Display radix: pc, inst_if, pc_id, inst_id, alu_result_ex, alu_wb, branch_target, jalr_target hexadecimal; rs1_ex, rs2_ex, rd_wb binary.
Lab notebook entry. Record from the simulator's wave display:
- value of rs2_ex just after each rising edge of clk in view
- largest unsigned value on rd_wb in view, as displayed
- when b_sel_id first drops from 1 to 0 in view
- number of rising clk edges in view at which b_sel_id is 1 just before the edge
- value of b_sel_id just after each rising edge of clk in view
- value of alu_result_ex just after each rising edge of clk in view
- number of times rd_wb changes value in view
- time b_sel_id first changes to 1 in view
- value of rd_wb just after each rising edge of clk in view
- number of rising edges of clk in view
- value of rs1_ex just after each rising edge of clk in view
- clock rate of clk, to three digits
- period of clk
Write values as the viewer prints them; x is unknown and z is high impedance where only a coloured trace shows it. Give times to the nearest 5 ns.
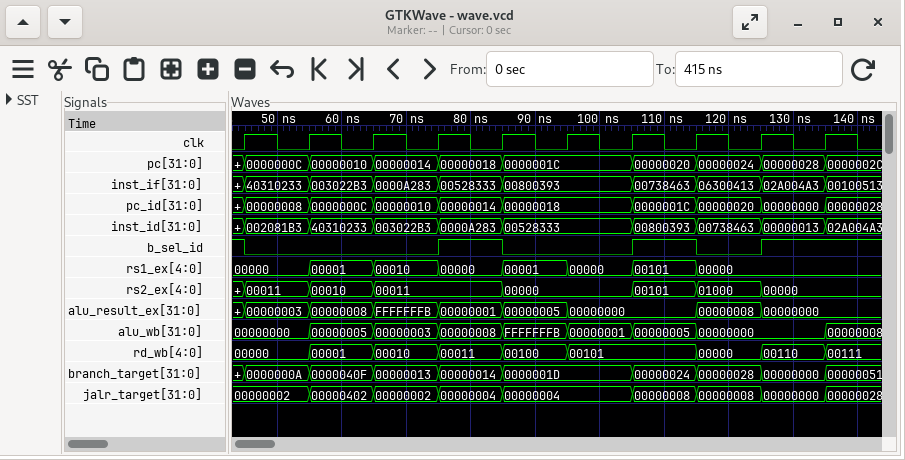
00011, 00010, 00011, 00011, 00000, 00000, 00101, 01000, 00000, 00000
00111
45 ns
4
0 0 0 1 0 0 1 0 1 1
00000003, 00000008, FFFFFFFB, 00000001, 00000005, 00000000, 00000000, 00000008, 00000000, 00000000
8
75 ns
00000, 00001, 00010, 00011, 00100, 00101, 00101, 00000, 00110, 00111
10
00000, 00001, 00010, 00000, 00001, 00000, 00101, 00000, 00000, 00000
100 MHz
10 ns
